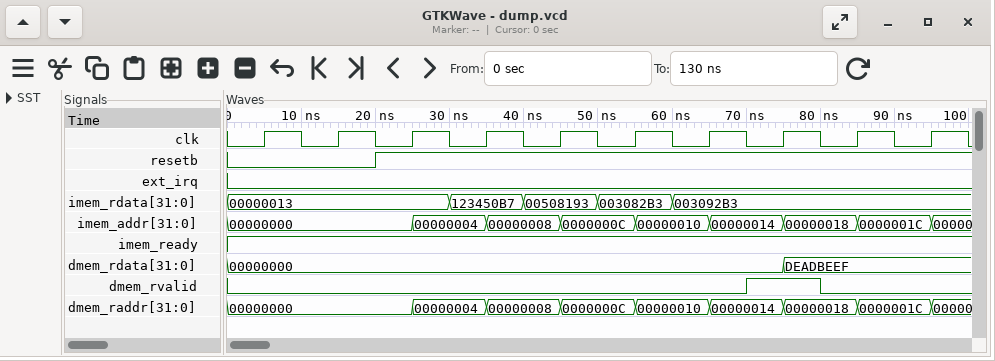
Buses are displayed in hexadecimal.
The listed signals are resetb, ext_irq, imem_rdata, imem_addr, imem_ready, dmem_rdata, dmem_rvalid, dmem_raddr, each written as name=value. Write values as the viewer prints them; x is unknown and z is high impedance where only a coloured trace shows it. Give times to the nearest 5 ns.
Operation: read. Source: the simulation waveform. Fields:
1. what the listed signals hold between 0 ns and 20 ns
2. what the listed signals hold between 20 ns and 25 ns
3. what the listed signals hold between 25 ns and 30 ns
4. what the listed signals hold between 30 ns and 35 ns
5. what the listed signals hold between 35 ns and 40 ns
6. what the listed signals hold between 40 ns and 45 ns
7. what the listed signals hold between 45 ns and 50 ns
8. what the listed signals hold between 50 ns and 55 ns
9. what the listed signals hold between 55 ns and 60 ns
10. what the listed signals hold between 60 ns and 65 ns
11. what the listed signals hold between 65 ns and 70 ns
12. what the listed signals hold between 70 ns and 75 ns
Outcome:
resetb=0, ext_irq=0, imem_rdata=00000013, imem_addr=00000000, imem_ready=1, dmem_rdata=00000000, dmem_rvalid=0, dmem_raddr=00000000
resetb=1, ext_irq=0, imem_rdata=00000013, imem_addr=00000000, imem_ready=1, dmem_rdata=00000000, dmem_rvalid=0, dmem_raddr=00000000
resetb=1, ext_irq=0, imem_rdata=00000013, imem_addr=00000004, imem_ready=1, dmem_rdata=00000000, dmem_rvalid=0, dmem_raddr=00000004
resetb=1, ext_irq=0, imem_rdata=123450B7, imem_addr=00000004, imem_ready=1, dmem_rdata=00000000, dmem_rvalid=0, dmem_raddr=00000004
resetb=1, ext_irq=0, imem_rdata=123450B7, imem_addr=00000008, imem_ready=1, dmem_rdata=00000000, dmem_rvalid=0, dmem_raddr=00000008
resetb=1, ext_irq=0, imem_rdata=00508193, imem_addr=00000008, imem_ready=1, dmem_rdata=00000000, dmem_rvalid=0, dmem_raddr=00000008
resetb=1, ext_irq=0, imem_rdata=00508193, imem_addr=0000000C, imem_ready=1, dmem_rdata=00000000, dmem_rvalid=0, dmem_raddr=0000000C
resetb=1, ext_irq=0, imem_rdata=003082B3, imem_addr=0000000C, imem_ready=1, dmem_rdata=00000000, dmem_rvalid=0, dmem_raddr=0000000C
resetb=1, ext_irq=0, imem_rdata=003082B3, imem_addr=00000010, imem_ready=1, dmem_rdata=00000000, dmem_rvalid=0, dmem_raddr=00000010
resetb=1, ext_irq=0, imem_rdata=003092B3, imem_addr=00000010, imem_ready=1, dmem_rdata=00000000, dmem_rvalid=0, dmem_raddr=00000010
resetb=1, ext_irq=0, imem_rdata=003092B3, imem_addr=00000014, imem_ready=1, dmem_rdata=00000000, dmem_rvalid=0, dmem_raddr=00000014
resetb=1, ext_irq=0, imem_rdata=003092B3, imem_addr=00000014, imem_ready=1, dmem_rdata=00000000, dmem_rvalid=1, dmem_raddr=00000014
